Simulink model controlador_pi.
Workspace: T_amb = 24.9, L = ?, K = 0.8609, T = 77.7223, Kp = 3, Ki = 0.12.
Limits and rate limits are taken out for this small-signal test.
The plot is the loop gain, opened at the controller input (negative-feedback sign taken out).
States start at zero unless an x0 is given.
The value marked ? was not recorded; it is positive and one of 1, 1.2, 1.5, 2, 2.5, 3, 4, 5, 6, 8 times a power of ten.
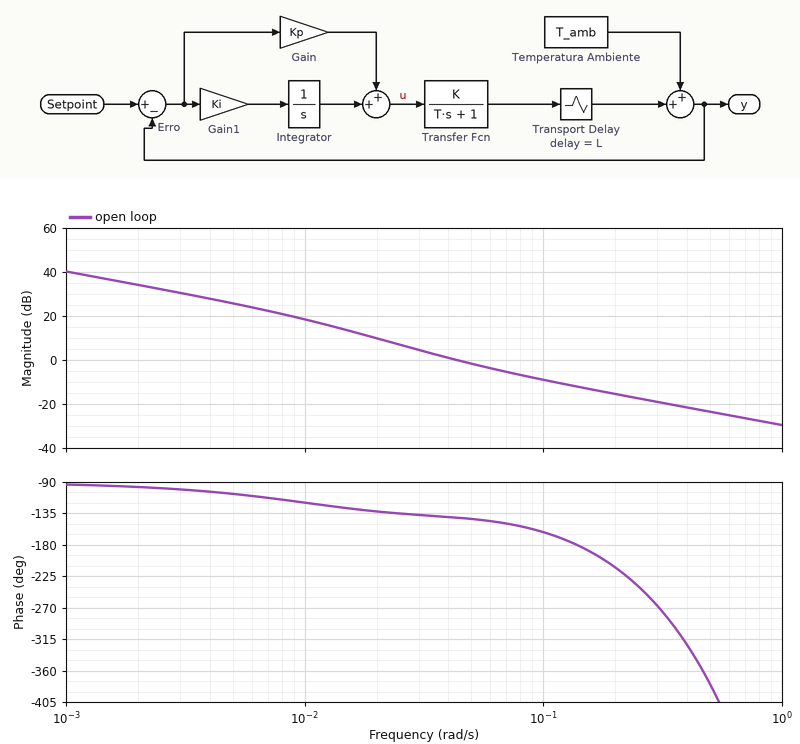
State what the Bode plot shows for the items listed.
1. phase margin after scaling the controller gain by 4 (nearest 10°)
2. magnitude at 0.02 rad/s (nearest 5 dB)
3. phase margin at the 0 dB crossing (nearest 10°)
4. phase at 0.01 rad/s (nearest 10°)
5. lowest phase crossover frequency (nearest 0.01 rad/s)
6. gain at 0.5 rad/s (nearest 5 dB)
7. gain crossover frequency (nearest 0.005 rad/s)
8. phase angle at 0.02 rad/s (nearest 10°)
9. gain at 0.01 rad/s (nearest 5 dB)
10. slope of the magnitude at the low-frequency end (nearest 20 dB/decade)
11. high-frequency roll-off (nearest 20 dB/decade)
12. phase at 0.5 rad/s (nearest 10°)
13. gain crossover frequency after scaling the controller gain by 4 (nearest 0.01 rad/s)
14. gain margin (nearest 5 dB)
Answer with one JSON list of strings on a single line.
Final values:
["0°", "10 dB", "40°", "-120°", "0.14 rad/s", "-25 dB", "0.045 rad/s", "-130°", "20 dB", "-20 dB/decade", "-20 dB/decade", "-380°", "0.14 rad/s", "10 dB"]
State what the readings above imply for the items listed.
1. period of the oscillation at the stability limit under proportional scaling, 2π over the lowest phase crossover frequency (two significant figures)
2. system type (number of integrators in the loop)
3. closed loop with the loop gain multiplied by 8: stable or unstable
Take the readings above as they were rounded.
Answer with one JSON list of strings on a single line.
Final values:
["45 s", "1", "unstable"]
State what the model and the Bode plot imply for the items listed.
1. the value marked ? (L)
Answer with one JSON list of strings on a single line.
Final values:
["10"]
